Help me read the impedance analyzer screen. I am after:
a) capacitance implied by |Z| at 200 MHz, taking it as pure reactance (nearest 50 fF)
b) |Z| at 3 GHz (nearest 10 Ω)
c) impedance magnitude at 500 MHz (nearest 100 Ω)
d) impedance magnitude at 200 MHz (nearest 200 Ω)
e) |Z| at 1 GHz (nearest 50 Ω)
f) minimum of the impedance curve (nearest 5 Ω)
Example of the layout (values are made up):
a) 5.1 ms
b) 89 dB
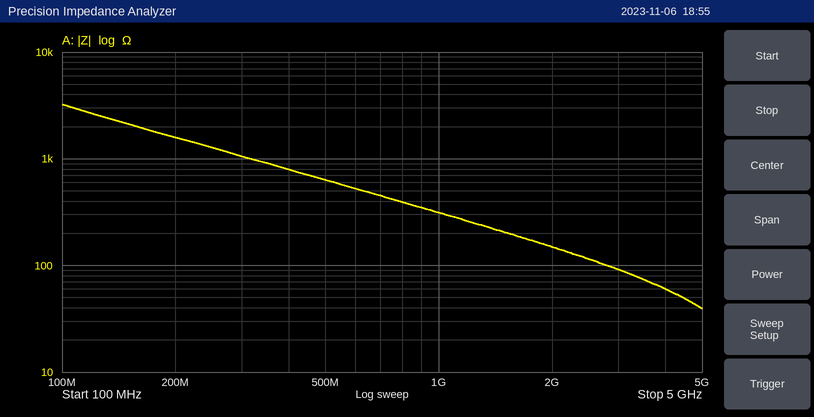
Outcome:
a) 500 fF
b) 90 Ω
c) 600 Ω
d) 1.6 kΩ
e) 300 Ω
f) 40 Ω
